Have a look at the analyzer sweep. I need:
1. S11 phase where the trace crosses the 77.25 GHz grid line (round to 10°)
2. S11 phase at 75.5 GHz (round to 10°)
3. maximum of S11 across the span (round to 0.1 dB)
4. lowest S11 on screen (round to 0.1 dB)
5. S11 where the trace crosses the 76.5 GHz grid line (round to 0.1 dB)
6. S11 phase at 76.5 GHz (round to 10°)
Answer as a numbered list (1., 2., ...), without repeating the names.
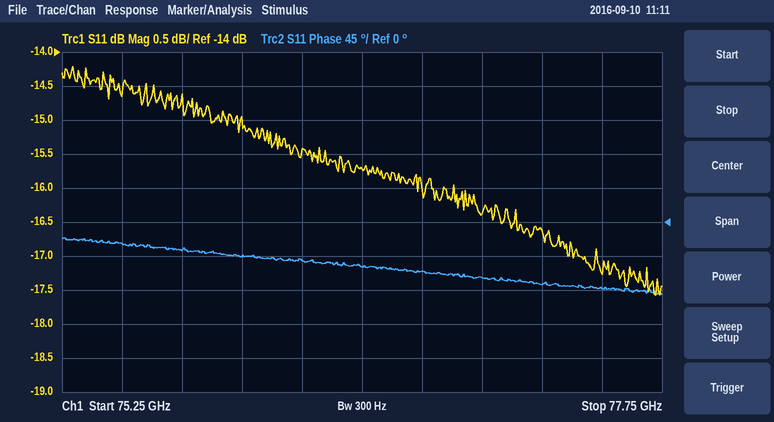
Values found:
1. -80°
2. -30°
3. -14.2 dB
4. -17.6 dB
5. -15.7 dB
6. -60°
